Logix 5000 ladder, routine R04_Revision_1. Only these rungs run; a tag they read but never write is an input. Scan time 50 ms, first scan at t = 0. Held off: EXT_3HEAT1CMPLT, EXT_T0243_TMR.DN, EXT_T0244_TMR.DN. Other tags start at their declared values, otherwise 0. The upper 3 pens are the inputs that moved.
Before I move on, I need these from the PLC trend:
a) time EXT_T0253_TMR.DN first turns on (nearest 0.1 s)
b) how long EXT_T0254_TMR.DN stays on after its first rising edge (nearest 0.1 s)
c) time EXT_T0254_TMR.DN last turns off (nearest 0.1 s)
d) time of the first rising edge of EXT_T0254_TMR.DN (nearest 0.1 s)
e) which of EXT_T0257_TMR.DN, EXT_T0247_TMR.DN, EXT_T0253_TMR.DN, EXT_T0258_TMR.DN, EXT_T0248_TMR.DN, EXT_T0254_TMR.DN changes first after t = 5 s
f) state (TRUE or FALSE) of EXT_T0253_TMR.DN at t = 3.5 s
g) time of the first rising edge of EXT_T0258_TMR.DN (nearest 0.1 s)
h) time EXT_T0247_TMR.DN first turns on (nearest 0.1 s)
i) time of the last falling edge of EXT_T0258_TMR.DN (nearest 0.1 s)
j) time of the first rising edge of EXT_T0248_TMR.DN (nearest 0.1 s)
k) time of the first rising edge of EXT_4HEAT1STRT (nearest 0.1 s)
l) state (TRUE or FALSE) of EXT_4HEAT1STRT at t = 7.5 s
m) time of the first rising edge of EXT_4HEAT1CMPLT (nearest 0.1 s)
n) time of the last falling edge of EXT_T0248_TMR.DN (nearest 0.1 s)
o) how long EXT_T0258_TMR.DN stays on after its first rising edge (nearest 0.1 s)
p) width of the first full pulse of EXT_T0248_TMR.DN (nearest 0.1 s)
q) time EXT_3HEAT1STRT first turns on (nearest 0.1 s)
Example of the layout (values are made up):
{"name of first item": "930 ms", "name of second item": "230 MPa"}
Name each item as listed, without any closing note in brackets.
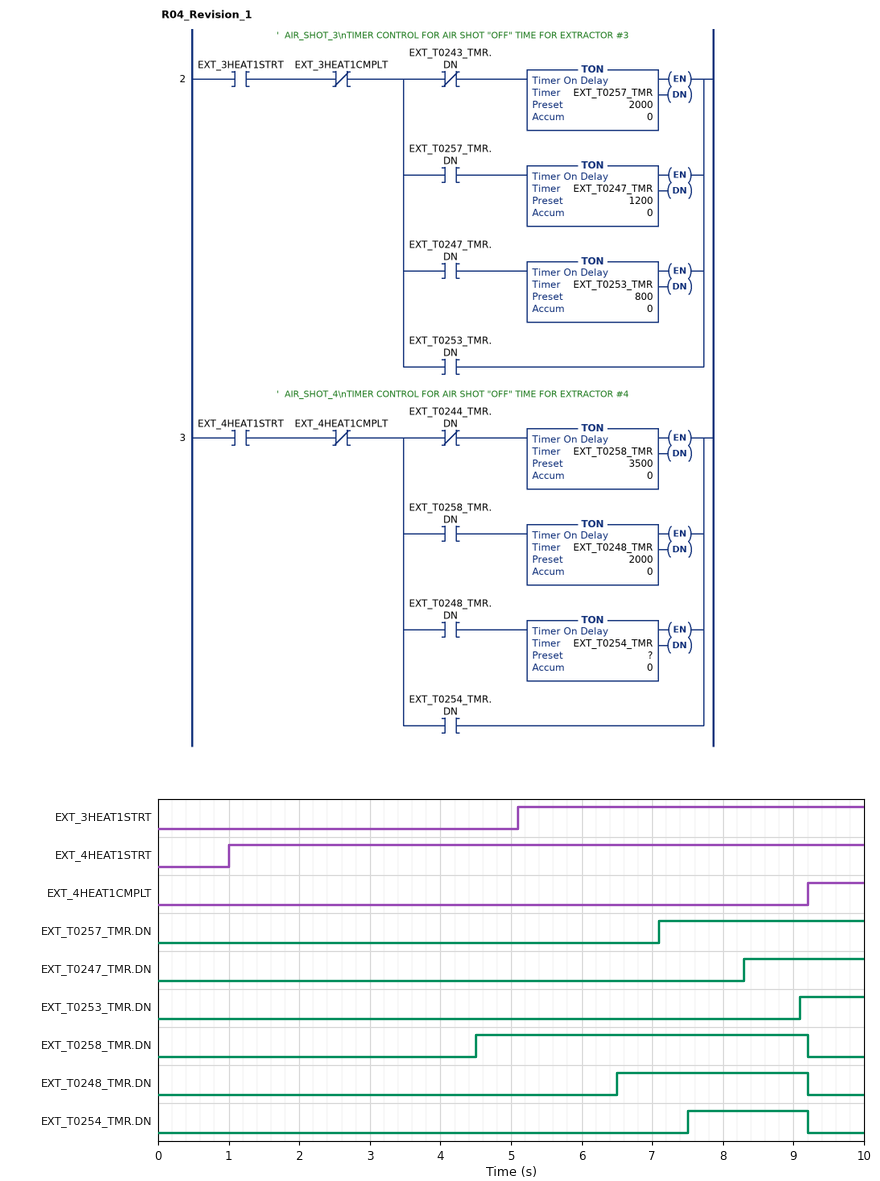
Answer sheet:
{"time EXT_T0253_TMR.DN first turns on": "9.1 s", "how long EXT_T0254_TMR.DN stays on after its first rising edge": "1.7 s", "time EXT_T0254_TMR.DN last turns off": "9.2 s", "time of the first rising edge of EXT_T0254_TMR.DN": "7.5 s", "which of EXT_T0257_TMR.DN, EXT_T0247_TMR.DN, EXT_T0253_TMR.DN, EXT_T0258_TMR.DN, EXT_T0248_TMR.DN, EXT_T0254_TMR.DN changes first after t = 5 s": "EXT_T0248_TMR.DN", "state (TRUE or FALSE) of EXT_T0253_TMR.DN at t = 3.5 s": "FALSE", "time of the first rising edge of EXT_T0258_TMR.DN": "4.5 s", "time EXT_T0247_TMR.DN first turns on": "8.3 s", "time of the last falling edge of EXT_T0258_TMR.DN": "9.2 s", "time of the first rising edge of EXT_T0248_TMR.DN": "6.5 s", "time of the first rising edge of EXT_4HEAT1STRT": "1.0 s", "state (TRUE or FALSE) of EXT_4HEAT1STRT at t = 7.5 s": "TRUE", "time of the first rising edge of EXT_4HEAT1CMPLT": "9.2 s", "time of the last falling edge of EXT_T0248_TMR.DN": "9.2 s", "how long EXT_T0258_TMR.DN stays on after its first rising edge": "4.7 s", "width of the first full pulse of EXT_T0248_TMR.DN": "2.7 s", "time EXT_3HEAT1STRT first turns on": "5.1 s"}
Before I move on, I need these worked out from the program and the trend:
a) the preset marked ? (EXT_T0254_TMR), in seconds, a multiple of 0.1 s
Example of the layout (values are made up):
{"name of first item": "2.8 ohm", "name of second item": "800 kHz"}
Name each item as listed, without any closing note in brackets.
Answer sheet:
{"the preset marked ? (EXT_T0254_TMR), in seconds, a multiple of 0.1 s": "1.0 s"}
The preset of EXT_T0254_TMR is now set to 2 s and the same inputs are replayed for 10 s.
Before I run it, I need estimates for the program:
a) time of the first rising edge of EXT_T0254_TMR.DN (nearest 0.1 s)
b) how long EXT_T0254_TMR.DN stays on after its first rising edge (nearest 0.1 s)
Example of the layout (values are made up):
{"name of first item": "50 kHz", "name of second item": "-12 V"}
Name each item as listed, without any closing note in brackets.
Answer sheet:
{"time of the first rising edge of EXT_T0254_TMR.DN": "8.5 s", "how long EXT_T0254_TMR.DN stays on after its first rising edge": "0.7 s"}
